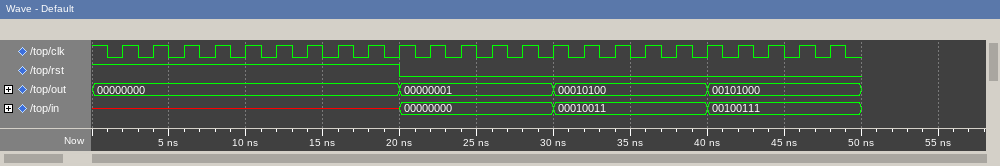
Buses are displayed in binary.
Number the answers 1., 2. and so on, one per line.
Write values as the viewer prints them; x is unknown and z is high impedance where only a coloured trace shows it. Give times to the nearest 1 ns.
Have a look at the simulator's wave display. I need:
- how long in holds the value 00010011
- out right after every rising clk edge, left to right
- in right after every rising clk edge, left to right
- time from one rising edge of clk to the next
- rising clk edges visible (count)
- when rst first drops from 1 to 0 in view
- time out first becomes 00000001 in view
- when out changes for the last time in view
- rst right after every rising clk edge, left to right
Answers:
1. 10 ns
2. 00000000, 00000000, 00000000, 00000000, 00000000, 00000000, 00000000, 00000000, 00000000, 00000001, 00000001, 00000001, 00000001, 00000001, 00010100, 00010100, 00010100, 00010100, 00010100, 00101000, 00101000, 00101000, 00101000, 00101000
3. x, x, x, x, x, x, x, x, x, 00000000, 00000000, 00000000, 00000000, 00000000, 00010011, 00010011, 00010011, 00010011, 00010011, 00100111, 00100111, 00100111, 00100111, 00100111
4. 2 ns
5. 24
6. 20 ns
7. 20 ns
8. 40 ns
9. 1 1 1 1 1 1 1 1 1 0 0 0 0 0 0 0 0 0 0 0 0 0 0 0
